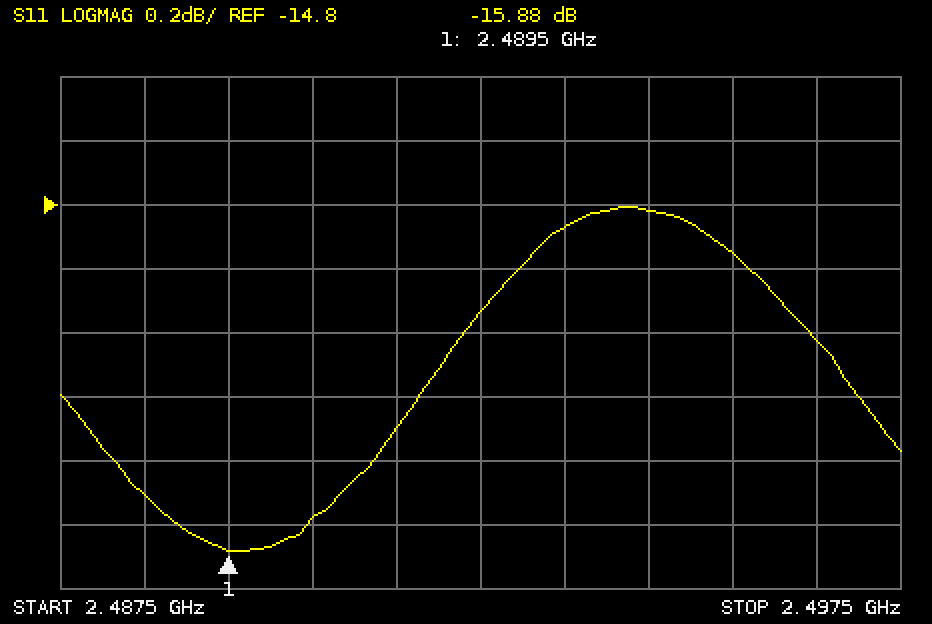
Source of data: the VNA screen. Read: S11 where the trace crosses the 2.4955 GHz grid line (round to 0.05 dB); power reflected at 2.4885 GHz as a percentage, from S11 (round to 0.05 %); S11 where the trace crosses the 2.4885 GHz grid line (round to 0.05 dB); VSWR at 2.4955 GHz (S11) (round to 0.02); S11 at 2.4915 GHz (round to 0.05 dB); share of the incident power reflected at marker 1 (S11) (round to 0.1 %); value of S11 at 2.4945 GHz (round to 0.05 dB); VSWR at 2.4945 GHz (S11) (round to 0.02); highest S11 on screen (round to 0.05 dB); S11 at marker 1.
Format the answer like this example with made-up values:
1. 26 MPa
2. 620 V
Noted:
1. -14.95 dB
2. 2.70 %
3. -15.70 dB
4. 1.44
5. -15.50 dB
6. 2.6 %
7. -14.80 dB
8. 1.44
9. -14.80 dB
10. -15.88 dB
